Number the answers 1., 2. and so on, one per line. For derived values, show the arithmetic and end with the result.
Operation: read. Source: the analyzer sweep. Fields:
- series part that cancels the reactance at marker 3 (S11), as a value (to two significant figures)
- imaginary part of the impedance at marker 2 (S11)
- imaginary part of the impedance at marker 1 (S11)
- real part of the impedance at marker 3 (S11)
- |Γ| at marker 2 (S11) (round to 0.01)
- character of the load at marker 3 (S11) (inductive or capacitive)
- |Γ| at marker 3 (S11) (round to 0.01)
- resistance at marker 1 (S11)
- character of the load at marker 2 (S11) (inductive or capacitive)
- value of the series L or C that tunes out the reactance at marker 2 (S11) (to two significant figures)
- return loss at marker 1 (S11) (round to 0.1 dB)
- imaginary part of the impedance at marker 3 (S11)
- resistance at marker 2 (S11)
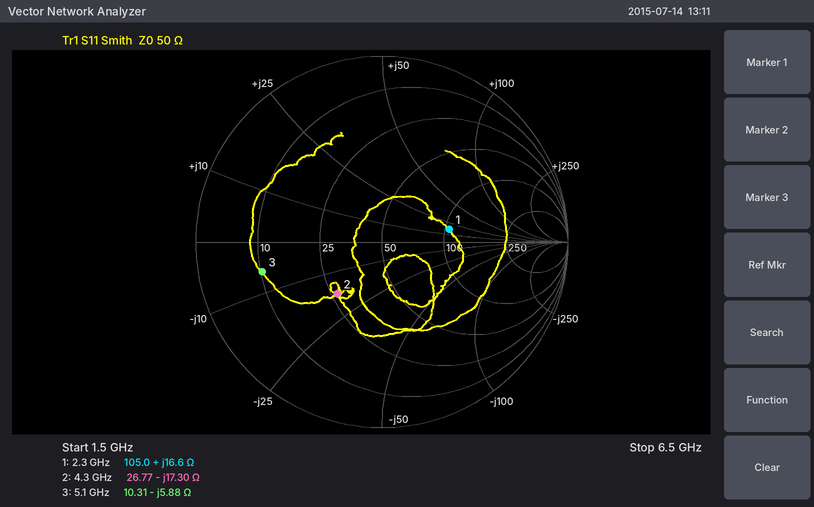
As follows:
1. L = 5.88 Ω/(2π × 5.1 GHz) ≈ 183 pH, so 180 pH to two significant figures
2. -17.30 Ω
3. +16.6 Ω
4. 10.31 Ω
5. 0.37
6. capacitive
7. 0.66
8. 105.0 Ω
9. capacitive
10. L = 17.3 Ω/(2π × 4.3 GHz) ≈ 640 pH
11. 8.7 dB
12. -5.88 Ω
13. 26.77 Ω
